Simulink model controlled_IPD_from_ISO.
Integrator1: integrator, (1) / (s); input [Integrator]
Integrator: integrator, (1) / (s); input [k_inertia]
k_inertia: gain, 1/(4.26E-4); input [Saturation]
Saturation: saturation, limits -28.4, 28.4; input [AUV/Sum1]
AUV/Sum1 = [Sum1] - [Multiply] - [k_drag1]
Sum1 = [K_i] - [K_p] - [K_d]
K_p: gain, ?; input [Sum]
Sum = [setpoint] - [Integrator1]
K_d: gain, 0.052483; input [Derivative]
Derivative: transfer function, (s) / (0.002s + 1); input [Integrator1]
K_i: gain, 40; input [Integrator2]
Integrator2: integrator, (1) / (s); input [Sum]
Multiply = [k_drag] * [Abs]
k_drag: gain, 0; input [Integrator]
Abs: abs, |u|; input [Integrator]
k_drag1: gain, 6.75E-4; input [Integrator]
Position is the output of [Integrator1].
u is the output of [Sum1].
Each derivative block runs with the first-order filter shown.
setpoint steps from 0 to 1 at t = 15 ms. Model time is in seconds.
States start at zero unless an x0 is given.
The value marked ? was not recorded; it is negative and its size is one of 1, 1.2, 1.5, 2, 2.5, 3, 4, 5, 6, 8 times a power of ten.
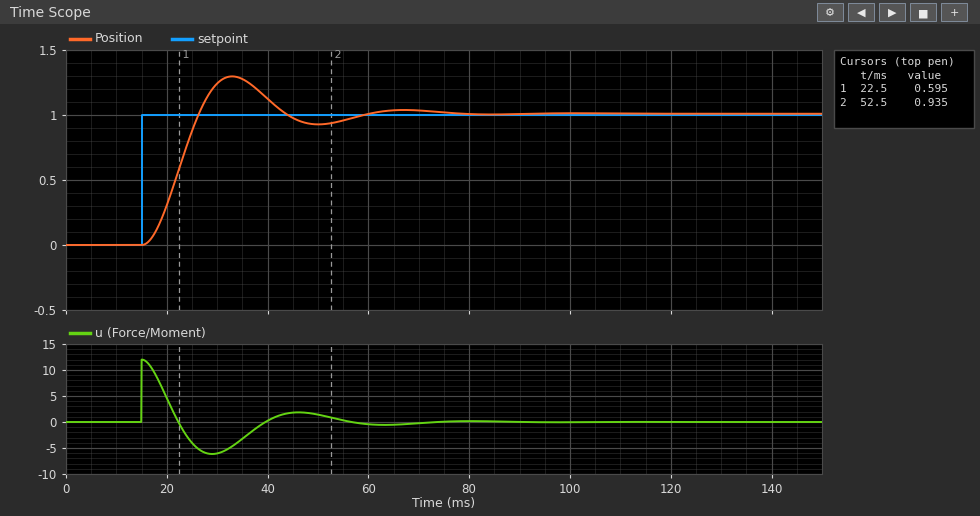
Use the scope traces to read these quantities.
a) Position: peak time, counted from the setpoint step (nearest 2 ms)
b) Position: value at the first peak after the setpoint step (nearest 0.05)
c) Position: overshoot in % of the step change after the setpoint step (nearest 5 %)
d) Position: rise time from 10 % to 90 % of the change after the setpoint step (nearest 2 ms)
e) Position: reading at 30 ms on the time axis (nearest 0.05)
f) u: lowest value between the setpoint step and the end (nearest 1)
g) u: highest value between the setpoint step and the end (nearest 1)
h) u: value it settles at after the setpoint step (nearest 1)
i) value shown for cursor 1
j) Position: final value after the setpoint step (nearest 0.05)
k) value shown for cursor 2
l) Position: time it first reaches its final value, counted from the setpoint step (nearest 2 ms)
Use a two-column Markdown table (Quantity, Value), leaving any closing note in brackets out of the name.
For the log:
| Quantity | Value |
|---|---|
| Position: peak time, counted from the setpoint step | 18 ms |
| Position: value at the first peak after the setpoint step | 1.30 |
| Position: overshoot in % of the step change after the setpoint step | 30 % |
| Position: rise time from 10 % to 90 % of the change after the setpoint step | 8 ms |
| Position: reading at 30 ms on the time axis | 1.25 |
| u: lowest value between the setpoint step and the end | -6 |
| u: highest value between the setpoint step and the end | 12 |
| u: value it settles at after the setpoint step | 0 |
| value shown for cursor 1 | 0.595 |
| Position: final value after the setpoint step | 1.00 |
| value shown for cursor 2 | 0.935 |
| Position: time it first reaches its final value, counted from the setpoint step | 12 ms |
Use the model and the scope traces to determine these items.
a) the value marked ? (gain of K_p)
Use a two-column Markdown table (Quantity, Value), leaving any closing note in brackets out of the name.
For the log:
| Quantity | Value |
|---|---|
| the value marked ? | -12 |
